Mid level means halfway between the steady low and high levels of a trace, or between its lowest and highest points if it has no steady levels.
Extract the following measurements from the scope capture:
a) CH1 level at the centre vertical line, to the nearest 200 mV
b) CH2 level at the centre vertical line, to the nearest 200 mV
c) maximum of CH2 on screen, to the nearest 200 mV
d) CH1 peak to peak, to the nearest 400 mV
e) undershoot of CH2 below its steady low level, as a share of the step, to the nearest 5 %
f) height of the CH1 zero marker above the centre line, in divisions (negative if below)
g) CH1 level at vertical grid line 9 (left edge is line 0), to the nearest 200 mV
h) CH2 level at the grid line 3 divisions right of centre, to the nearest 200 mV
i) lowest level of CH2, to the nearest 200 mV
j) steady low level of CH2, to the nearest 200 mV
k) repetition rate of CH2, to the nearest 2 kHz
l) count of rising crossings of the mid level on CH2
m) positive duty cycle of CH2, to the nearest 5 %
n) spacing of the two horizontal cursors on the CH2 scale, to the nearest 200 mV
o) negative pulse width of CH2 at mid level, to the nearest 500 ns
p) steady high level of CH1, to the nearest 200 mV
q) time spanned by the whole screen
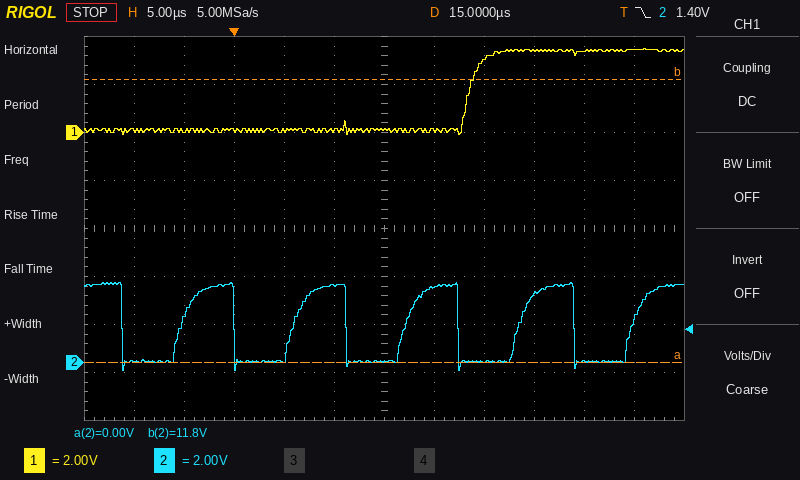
200 mV
0.0 V
3.4 V
3.6 V
10 %
+2.0 div
3.4 V
2.8 V
-400 mV
0.0 V
88 kHz
5
45 %
11.8 V
6.0 µs
3.4 V
60 µs
